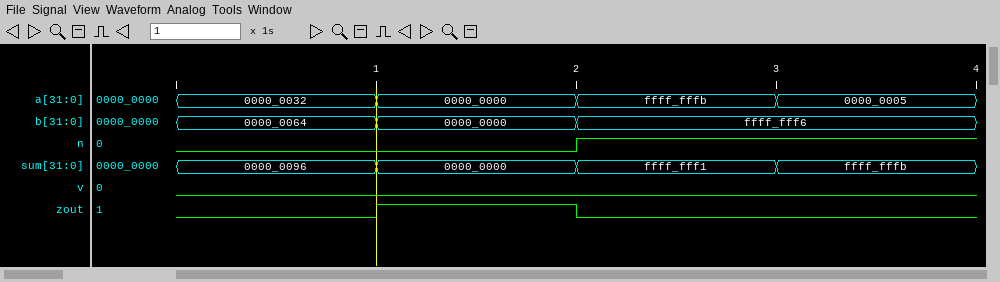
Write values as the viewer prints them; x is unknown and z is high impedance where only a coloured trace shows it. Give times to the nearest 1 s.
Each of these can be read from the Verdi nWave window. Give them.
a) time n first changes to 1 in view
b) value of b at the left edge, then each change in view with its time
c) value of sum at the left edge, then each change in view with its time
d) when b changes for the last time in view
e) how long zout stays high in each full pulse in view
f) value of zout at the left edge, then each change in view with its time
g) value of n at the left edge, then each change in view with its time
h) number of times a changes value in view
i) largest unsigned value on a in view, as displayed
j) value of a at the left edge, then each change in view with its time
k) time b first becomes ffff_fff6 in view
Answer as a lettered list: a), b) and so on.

a) 2 s
b) 0000_0064, 0000_0000 at 1 s, ffff_fff6 at 2 s
c) 0000_0096, 0000_0000 at 1 s, ffff_fff1 at 2 s, ffff_fffb at 3 s
d) 2 s
e) 1 s
f) 0, 1 at 1 s, 0 at 2 s
g) 0, 1 at 2 s
h) 3
i) ffff_fffb
j) 0000_0032, 0000_0000 at 1 s, ffff_fffb at 2 s, 0000_0005 at 3 s
k) 2 s
